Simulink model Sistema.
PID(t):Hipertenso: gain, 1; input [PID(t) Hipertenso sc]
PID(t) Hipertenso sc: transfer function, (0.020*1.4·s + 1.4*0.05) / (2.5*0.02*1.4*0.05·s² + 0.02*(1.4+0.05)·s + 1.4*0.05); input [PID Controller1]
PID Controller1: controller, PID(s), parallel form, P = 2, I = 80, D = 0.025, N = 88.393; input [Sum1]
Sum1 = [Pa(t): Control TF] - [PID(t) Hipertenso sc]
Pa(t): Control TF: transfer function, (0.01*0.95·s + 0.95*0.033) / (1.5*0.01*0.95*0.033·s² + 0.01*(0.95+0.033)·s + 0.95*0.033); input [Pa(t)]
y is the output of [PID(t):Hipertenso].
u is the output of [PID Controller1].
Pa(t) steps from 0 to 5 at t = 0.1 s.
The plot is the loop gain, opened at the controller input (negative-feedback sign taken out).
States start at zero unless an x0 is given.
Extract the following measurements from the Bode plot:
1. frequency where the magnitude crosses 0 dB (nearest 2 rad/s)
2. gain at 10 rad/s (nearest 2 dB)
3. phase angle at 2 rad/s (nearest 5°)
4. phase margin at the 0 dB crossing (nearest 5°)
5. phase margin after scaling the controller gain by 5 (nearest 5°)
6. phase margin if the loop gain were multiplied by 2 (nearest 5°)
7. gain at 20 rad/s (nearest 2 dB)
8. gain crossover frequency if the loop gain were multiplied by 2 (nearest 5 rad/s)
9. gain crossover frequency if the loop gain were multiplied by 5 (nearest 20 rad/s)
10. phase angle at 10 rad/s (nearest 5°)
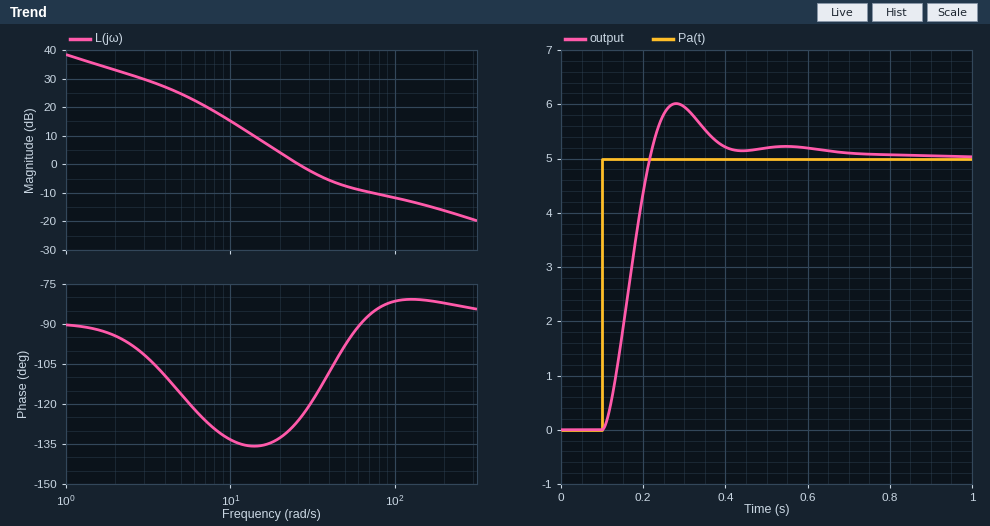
26 rad/s
16 dB
-95°
55°
100°
75°
4 dB
40 rad/s
140 rad/s
-135°
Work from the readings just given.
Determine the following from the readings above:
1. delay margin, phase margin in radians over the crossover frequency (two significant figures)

0.037 s
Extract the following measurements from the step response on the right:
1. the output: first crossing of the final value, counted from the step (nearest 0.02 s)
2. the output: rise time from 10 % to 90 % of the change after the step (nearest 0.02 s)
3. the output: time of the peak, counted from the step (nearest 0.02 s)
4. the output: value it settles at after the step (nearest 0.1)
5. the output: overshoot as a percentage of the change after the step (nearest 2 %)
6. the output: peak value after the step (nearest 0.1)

0.12 s
0.08 s
0.18 s
5.0
20 %
6.0
